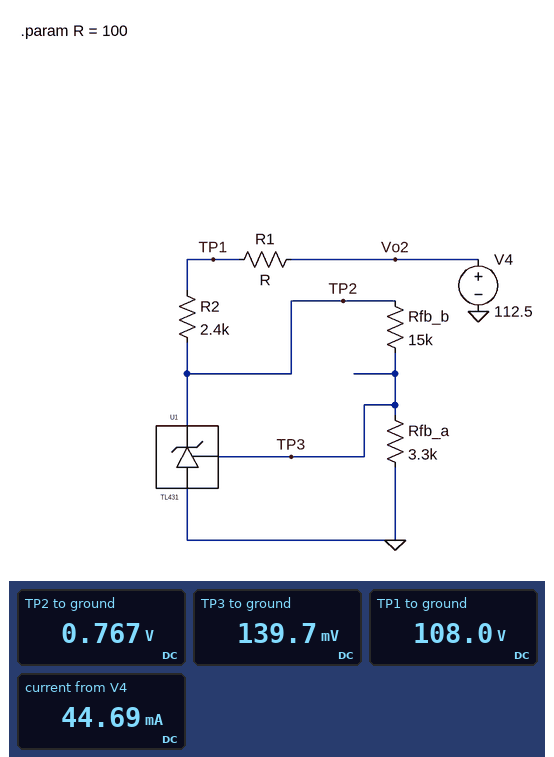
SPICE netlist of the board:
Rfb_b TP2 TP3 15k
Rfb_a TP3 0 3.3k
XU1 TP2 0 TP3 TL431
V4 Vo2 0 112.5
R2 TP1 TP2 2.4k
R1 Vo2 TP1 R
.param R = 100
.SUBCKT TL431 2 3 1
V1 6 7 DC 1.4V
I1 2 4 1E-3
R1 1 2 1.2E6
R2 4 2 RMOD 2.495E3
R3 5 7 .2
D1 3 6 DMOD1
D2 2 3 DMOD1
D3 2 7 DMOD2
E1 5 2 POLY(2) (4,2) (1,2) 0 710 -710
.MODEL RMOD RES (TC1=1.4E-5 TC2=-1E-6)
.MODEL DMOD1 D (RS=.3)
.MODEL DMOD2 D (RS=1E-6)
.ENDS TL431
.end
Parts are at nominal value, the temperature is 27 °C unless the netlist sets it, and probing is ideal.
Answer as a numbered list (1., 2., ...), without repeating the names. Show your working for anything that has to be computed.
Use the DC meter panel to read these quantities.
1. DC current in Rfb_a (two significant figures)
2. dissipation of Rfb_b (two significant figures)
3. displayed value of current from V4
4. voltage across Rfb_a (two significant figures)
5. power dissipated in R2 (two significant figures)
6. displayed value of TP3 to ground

1. (139.7 mV) / 3.3 kΩ = 42 µA
2. (767 mV - 139.7 mV)^2 / 15 kΩ = 26 µW
3. 44.69 mA
4. 139.7 mV = 140 mV
5. (108 V - 767 mV)^2 / 2.4 kΩ = 4.8 W
6. 139.7 mV
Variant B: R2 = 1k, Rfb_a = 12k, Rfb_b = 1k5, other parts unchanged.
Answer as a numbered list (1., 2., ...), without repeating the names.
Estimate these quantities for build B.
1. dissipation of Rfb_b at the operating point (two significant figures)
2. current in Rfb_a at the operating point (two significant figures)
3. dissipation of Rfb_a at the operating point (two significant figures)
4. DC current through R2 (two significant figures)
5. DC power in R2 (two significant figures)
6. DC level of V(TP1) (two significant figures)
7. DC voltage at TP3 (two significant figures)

1. 5.3 µW
2. 60 µA
3. 43 µW
4. 100 mA
5. 10 W
6. 100 V
7. 720 mV
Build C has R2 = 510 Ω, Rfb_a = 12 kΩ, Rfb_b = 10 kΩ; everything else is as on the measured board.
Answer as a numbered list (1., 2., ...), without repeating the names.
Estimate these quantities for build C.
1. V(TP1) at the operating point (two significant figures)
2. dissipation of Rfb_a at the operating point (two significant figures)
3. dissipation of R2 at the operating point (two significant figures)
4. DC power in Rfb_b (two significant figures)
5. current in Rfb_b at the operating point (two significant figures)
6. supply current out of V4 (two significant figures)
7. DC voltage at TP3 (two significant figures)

1. 94 V
2. 18 µW
3. 17 W
4. 15 µW
5. 38 µA
6. 180 mA
7. 460 mV
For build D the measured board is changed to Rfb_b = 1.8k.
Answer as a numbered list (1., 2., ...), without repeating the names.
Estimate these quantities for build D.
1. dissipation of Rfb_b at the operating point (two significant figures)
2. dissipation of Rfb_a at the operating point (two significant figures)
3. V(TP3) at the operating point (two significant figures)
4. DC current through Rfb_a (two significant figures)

1. 41 µW
2. 75 µW
3. 500 mV
4. 150 µA
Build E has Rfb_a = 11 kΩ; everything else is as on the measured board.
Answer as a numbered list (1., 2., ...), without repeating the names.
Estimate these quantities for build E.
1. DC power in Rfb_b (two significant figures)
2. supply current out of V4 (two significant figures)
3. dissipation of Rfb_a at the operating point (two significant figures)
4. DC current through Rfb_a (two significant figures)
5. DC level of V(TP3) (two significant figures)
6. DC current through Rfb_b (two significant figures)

1. 13 µW
2. 45 mA
3. 9.7 µW
4. 30 µA
5. 330 mV
6. 29 µA
